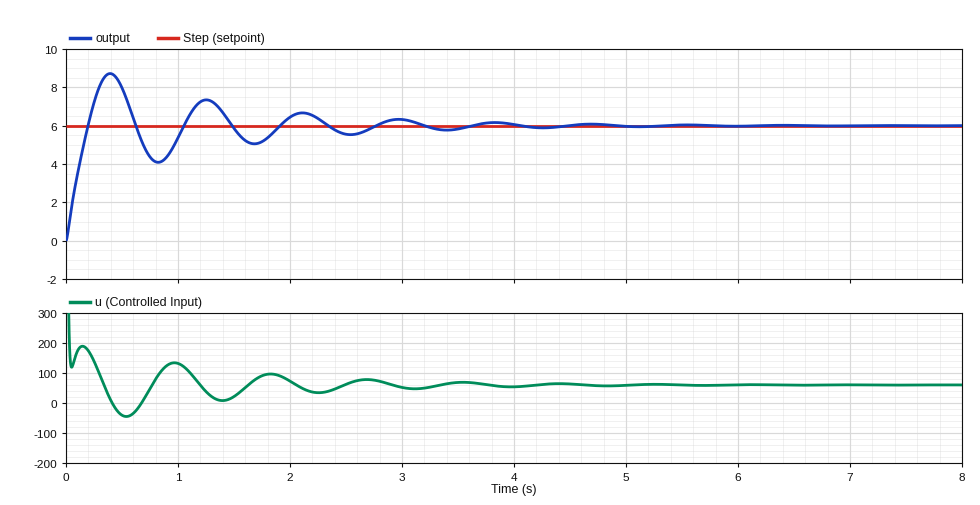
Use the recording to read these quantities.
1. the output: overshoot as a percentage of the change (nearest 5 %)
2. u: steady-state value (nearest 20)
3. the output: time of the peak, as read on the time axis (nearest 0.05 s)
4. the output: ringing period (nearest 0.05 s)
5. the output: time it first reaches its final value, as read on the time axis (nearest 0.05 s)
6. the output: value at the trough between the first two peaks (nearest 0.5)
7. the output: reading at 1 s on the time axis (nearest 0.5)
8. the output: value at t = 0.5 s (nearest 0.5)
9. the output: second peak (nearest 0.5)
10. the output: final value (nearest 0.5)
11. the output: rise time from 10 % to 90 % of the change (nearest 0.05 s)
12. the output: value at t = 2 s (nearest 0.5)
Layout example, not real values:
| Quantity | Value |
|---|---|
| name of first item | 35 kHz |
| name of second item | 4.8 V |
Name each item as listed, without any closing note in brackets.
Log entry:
| Quantity | Value |
|---|---|
| the output: overshoot as a percentage of the change | 45 % |
| u: steady-state value | 60 |
| the output: time of the peak, as read on the time axis | 0.40 s |
| the output: ringing period | 0.85 s |
| the output: time it first reaches its final value, as read on the time axis | 0.20 s |
| the output: value at the trough between the first two peaks | 4.0 |
| the output: reading at 1 s on the time axis | 5.5 |
| the output: value at t = 0.5 s | 8.0 |
| the output: second peak | 7.5 |
| the output: final value | 6.0 |
| the output: rise time from 10 % to 90 % of the change | 0.15 s |
| the output: value at t = 2 s | 6.5 |
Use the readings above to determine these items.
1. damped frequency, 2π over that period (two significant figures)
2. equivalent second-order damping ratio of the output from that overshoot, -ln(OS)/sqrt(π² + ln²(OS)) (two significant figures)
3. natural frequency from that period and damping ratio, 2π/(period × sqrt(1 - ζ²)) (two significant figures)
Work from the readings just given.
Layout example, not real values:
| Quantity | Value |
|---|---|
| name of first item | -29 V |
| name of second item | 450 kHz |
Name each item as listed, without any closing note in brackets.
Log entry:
| Quantity | Value |
|---|---|
| damped frequency, 2π over that period | 7.4 rad/s |
| equivalent second-order damping ratio of the output from that overshoot, -ln(OS)/sqrt(π² + ln²(OS)) | 0.25 |
| natural frequency from that period and damping ratio, 2π/(period × sqrt(1 - ζ²)) | 7.6 rad/s |
